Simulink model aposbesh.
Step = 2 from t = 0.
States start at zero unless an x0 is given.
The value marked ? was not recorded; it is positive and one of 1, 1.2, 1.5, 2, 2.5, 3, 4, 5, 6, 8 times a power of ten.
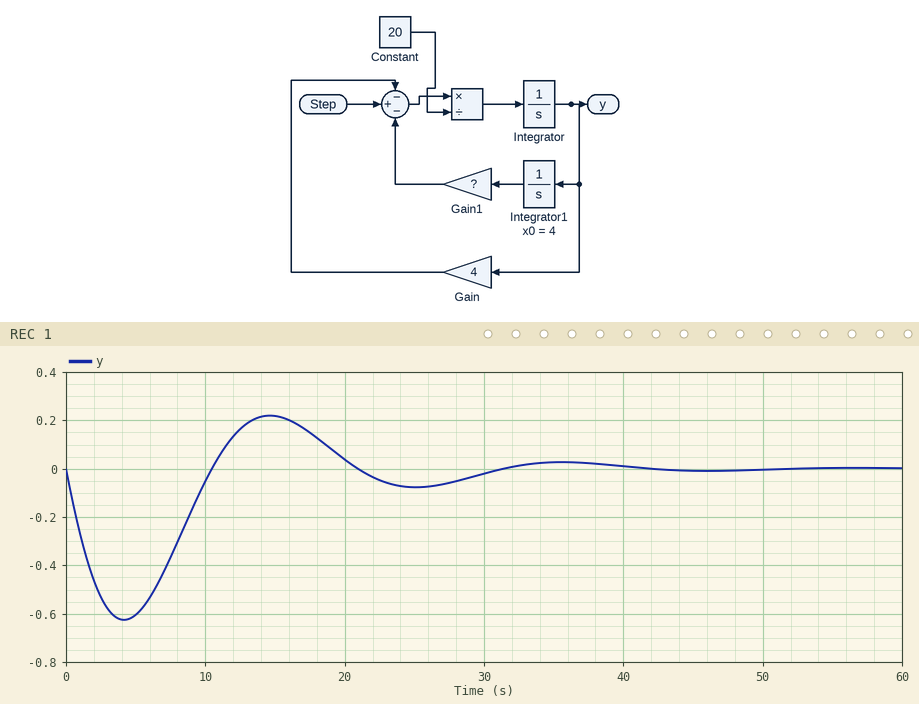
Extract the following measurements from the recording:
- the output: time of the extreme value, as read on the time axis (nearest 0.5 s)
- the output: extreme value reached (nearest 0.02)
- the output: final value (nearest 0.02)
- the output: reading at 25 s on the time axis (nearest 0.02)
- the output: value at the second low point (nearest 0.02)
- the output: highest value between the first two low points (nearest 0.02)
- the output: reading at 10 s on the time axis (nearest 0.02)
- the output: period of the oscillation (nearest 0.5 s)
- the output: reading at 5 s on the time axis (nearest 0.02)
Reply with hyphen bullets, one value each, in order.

- 4.0 s
- -0.62
- 0.00
- -0.08
- -0.08
- 0.22
- -0.06
- 21.0 s
- -0.60
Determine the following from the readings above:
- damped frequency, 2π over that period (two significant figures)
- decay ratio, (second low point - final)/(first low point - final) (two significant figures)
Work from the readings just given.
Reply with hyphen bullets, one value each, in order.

- 0.30 rad/s
- 0.13
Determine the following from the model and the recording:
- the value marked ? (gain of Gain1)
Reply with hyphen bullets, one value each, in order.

- 2
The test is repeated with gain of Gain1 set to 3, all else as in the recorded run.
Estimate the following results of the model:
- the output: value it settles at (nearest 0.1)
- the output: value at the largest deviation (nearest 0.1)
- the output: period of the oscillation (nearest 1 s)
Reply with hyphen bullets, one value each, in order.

- 0.0
- -0.9
- 17 s
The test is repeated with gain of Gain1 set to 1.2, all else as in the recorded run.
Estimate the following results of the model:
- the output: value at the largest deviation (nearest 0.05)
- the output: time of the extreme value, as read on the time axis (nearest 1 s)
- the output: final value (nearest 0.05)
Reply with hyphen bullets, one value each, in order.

- -0.35
- 5 s
- 0.00
